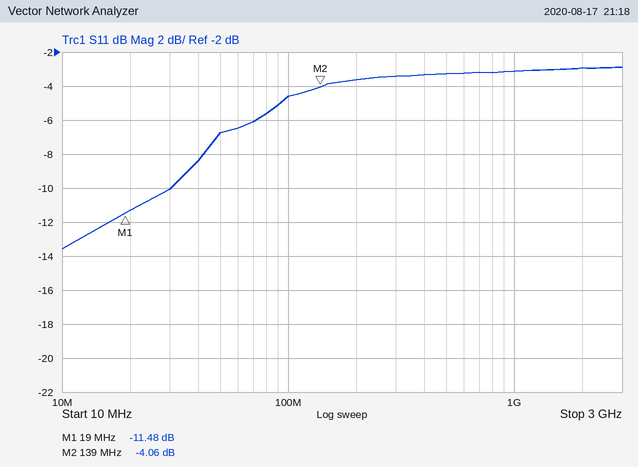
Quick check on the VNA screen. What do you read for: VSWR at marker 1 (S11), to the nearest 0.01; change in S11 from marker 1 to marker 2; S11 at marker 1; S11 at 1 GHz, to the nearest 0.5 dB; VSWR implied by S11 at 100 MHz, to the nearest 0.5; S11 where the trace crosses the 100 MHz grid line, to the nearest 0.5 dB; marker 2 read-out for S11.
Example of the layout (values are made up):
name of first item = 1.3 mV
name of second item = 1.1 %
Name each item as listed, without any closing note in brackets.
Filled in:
VSWR at marker 1 (S11), to the nearest 0.01 = 1.73
change in S11 from marker 1 to marker 2 = 7.42 dB
S11 at marker 1 = -11.48 dB
S11 at 1 GHz, to the nearest 0.5 dB = -3.0 dB
VSWR implied by S11 at 100 MHz, to the nearest 0.5 = 4.0
S11 where the trace crosses the 100 MHz grid line, to the nearest 0.5 dB = -4.5 dB
marker 2 read-out for S11 = -4.06 dB
